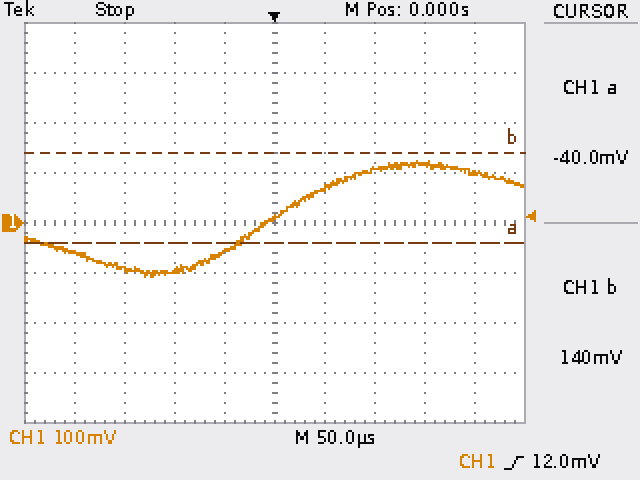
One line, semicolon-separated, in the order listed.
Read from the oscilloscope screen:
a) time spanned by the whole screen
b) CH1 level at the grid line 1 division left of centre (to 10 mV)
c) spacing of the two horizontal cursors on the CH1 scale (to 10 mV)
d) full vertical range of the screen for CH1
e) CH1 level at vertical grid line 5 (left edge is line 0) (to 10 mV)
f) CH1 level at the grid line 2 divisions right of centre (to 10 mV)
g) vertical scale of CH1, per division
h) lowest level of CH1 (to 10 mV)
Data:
500 µs; -60 mV; 180 mV; 800 mV; 10 mV; 110 mV; 100 mV; -110 mV
